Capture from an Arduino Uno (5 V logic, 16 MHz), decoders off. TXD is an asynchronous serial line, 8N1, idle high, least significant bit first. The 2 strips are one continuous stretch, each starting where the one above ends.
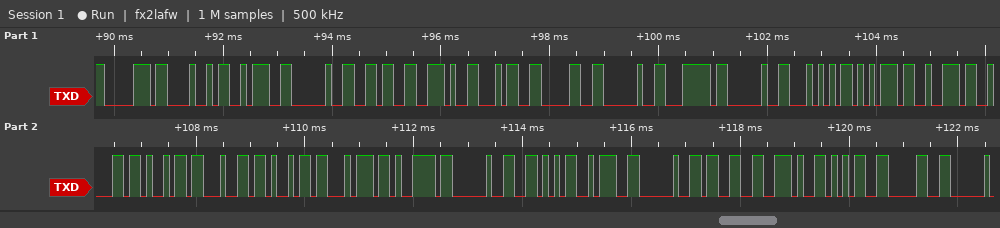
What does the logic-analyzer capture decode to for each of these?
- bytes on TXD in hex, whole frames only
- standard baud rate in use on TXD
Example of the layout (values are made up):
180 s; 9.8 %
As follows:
70 48 3A 20 36 2E 34 30 20 7C 20 54 75 72 62 69 64 69 74 79 20 56 3A 20 33 2E 35 30; 9600 baud
